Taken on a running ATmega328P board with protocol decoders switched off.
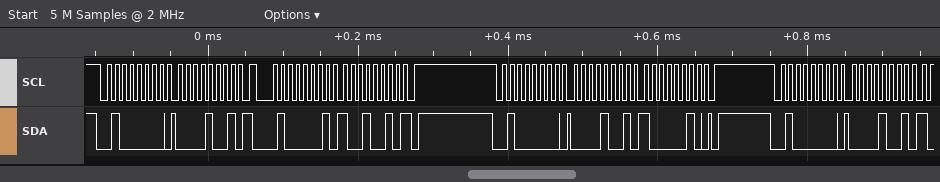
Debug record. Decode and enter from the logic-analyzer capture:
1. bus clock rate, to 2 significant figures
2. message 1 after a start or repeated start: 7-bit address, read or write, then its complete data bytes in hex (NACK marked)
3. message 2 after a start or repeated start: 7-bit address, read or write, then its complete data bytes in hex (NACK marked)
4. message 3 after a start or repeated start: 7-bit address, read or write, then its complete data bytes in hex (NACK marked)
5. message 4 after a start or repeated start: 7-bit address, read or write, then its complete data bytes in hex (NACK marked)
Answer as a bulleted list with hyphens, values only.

- 100 kHz
- 0x20 write: 09
- 0x20 read: 92 NACK
- 0x20 write: 09 82
- 0x20 write: 09
